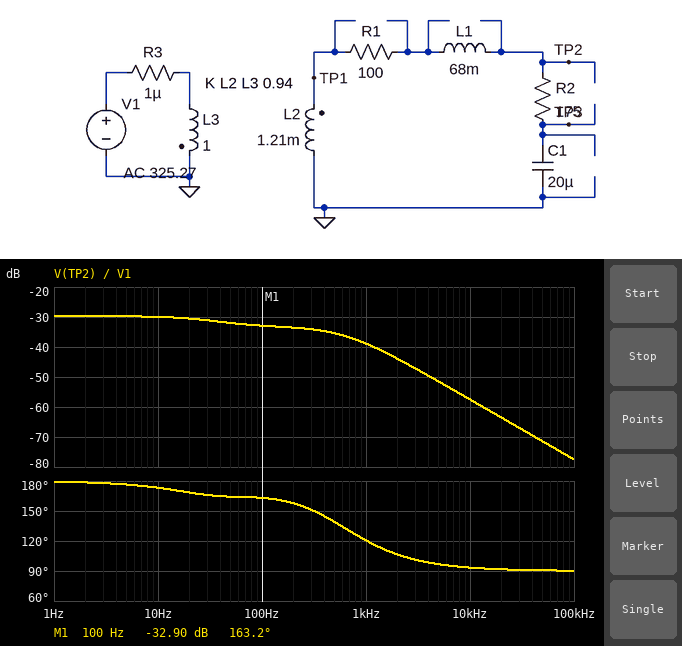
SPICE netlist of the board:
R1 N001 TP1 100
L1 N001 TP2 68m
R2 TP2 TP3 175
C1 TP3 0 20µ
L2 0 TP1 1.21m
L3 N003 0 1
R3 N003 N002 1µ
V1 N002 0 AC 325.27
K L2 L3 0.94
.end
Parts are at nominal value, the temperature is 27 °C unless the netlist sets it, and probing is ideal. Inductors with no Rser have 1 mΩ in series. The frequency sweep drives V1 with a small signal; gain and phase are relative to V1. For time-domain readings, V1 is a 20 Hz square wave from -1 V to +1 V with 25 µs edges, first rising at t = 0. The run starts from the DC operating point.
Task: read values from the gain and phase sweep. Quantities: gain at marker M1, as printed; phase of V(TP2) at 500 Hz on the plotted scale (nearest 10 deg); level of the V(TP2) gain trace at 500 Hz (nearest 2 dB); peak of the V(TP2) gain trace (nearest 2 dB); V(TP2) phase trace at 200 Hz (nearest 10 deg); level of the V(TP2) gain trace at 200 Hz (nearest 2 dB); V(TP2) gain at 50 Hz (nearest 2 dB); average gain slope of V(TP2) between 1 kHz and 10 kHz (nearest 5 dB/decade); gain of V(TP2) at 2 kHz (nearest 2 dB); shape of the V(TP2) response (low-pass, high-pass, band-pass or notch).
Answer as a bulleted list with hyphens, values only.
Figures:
- -32.90 dB
- 140 deg
- -36 dB
- -30 dB
- 160 deg
- -34 dB
- -32 dB
- -20 dB/decade
- -44 dB
- low-pass
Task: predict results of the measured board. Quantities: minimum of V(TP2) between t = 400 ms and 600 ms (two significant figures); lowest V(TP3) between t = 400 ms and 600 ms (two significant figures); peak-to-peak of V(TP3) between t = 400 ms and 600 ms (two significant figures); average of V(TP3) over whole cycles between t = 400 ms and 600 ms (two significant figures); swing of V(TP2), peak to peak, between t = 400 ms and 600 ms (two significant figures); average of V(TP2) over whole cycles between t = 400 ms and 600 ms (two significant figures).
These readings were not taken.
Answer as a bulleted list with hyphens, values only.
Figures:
- -65 mV
- -65 mV
- 64 mV
- -33 mV
- 65 mV
- -33 mV
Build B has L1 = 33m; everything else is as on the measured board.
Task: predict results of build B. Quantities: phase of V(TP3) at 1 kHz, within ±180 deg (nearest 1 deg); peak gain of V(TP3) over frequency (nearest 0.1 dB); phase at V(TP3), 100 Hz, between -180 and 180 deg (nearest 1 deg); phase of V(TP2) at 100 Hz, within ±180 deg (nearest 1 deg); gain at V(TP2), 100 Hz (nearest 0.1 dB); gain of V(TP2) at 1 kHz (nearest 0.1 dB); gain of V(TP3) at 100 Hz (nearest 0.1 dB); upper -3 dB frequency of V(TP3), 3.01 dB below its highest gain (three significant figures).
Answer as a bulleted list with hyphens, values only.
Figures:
- 54 deg
- -29.7 dB
- 102 deg
- 168 deg
- -33.0 dB
- -35.5 dB
- -40.7 dB
- 29.6 Hz
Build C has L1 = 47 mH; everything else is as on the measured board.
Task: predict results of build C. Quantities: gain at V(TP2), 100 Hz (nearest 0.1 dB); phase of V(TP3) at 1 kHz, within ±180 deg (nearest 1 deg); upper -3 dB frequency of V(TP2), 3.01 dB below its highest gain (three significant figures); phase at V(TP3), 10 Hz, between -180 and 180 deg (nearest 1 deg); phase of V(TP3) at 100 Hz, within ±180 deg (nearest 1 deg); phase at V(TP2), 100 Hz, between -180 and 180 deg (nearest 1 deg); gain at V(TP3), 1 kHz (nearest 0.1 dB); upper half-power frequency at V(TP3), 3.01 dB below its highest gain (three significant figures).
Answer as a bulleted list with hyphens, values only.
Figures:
- -33.0 dB
- 44 deg
- 78.8 Hz
- 161 deg
- 100 deg
- 166 deg
- -63.7 dB
- 29.9 Hz
